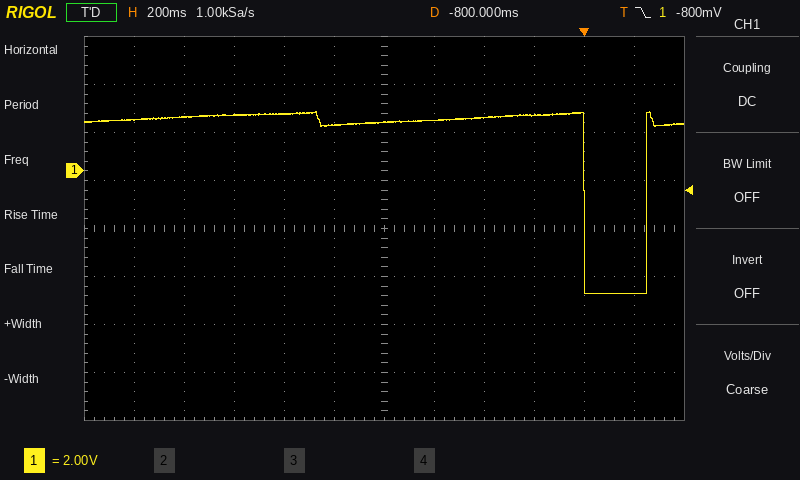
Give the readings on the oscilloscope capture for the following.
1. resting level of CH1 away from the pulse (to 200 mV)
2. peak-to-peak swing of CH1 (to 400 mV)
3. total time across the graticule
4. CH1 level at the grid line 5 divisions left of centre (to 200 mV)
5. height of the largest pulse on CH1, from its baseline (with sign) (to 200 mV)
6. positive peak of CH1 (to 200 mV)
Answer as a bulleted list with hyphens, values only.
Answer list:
- 2.2 V
- 7.6 V
- 2.4 s
- 2.2 V
- -7.4 V
- 2.4 V
